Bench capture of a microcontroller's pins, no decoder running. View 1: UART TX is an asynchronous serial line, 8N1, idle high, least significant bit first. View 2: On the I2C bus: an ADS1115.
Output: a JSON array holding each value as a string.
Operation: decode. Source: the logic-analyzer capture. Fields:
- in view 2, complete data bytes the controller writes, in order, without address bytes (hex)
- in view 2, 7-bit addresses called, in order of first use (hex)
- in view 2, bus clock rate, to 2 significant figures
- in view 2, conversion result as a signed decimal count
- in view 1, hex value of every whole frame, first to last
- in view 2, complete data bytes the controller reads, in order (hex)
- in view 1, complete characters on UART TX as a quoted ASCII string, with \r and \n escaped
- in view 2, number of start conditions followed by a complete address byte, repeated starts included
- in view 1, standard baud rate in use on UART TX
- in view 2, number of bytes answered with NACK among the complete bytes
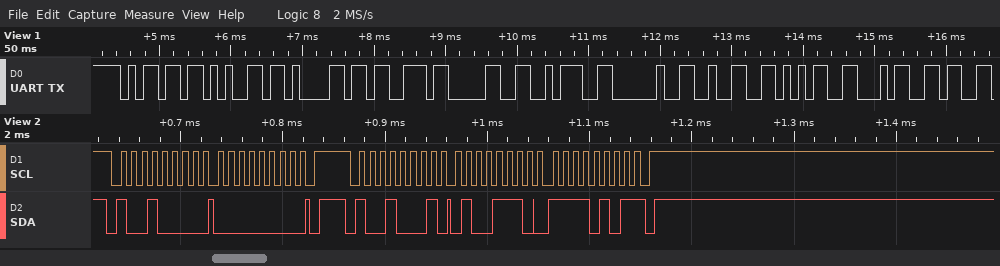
["00", "0x48", "100 kHz", "20213", "0x6D 0x65 0x61 0x73 0x30 0x3A 0x20 0x32 0x35 0x34", "4E F5", "\"meas0: 254\"", "2", "9600 baud", "1"]
